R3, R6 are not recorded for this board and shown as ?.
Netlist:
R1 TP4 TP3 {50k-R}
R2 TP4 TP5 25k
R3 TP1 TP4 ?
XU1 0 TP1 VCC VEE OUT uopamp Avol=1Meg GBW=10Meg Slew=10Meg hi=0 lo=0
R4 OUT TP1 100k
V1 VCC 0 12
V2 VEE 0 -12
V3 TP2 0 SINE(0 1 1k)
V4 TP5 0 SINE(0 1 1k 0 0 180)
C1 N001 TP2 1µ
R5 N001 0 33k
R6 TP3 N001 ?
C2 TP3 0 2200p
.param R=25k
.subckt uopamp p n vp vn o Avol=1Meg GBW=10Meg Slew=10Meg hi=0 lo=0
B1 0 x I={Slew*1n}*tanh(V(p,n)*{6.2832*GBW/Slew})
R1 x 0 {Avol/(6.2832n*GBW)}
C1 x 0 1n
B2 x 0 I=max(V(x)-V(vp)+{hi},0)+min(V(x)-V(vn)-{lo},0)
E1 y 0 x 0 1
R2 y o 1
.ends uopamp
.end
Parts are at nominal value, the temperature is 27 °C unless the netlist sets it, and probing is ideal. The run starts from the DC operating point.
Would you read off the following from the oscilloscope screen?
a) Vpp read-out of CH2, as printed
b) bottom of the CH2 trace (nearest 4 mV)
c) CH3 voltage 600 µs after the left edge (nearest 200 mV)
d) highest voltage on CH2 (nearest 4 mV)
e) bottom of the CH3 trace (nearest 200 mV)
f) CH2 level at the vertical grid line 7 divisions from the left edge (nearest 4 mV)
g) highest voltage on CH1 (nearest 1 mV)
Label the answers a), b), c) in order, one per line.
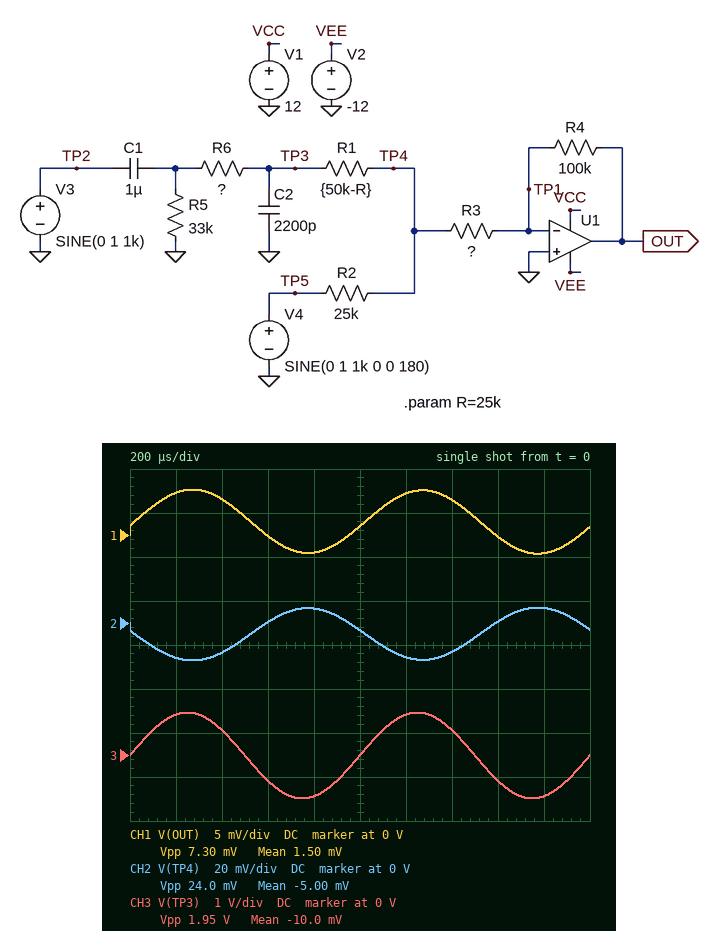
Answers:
a) 24.0 mV
b) -16 mV
c) -600 mV
d) 8 mV
e) -1.0 V
f) -12 mV
g) 5 mV
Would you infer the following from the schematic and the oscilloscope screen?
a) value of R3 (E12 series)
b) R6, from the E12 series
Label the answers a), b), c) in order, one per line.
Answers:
a) 330 kΩ
b) 560 Ω
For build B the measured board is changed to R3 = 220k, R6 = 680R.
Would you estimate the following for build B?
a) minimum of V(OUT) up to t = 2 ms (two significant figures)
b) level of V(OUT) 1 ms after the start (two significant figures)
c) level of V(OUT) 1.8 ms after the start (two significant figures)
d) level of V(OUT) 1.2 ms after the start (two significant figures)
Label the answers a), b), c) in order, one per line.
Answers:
a) -4.1 mV
b) 1.8 mV
c) -3.9 mV
d) 8.0 mV
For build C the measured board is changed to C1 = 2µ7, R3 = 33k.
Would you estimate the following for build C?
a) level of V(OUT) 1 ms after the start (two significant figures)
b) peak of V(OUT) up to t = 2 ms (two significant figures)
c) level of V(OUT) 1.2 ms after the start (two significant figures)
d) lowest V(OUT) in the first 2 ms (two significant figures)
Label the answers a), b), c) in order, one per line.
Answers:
a) 8.1 mV
b) 30 mV
c) 29 mV
d) -21 mV
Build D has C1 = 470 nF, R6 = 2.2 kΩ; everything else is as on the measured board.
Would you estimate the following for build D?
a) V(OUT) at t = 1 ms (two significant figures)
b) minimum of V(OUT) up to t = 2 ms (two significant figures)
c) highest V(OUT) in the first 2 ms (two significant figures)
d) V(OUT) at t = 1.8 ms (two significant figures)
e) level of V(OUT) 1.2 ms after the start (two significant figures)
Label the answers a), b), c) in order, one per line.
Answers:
a) 3.5 mV
b) -10 mV
c) 16 mV
d) -9.4 mV
e) 15 mV
